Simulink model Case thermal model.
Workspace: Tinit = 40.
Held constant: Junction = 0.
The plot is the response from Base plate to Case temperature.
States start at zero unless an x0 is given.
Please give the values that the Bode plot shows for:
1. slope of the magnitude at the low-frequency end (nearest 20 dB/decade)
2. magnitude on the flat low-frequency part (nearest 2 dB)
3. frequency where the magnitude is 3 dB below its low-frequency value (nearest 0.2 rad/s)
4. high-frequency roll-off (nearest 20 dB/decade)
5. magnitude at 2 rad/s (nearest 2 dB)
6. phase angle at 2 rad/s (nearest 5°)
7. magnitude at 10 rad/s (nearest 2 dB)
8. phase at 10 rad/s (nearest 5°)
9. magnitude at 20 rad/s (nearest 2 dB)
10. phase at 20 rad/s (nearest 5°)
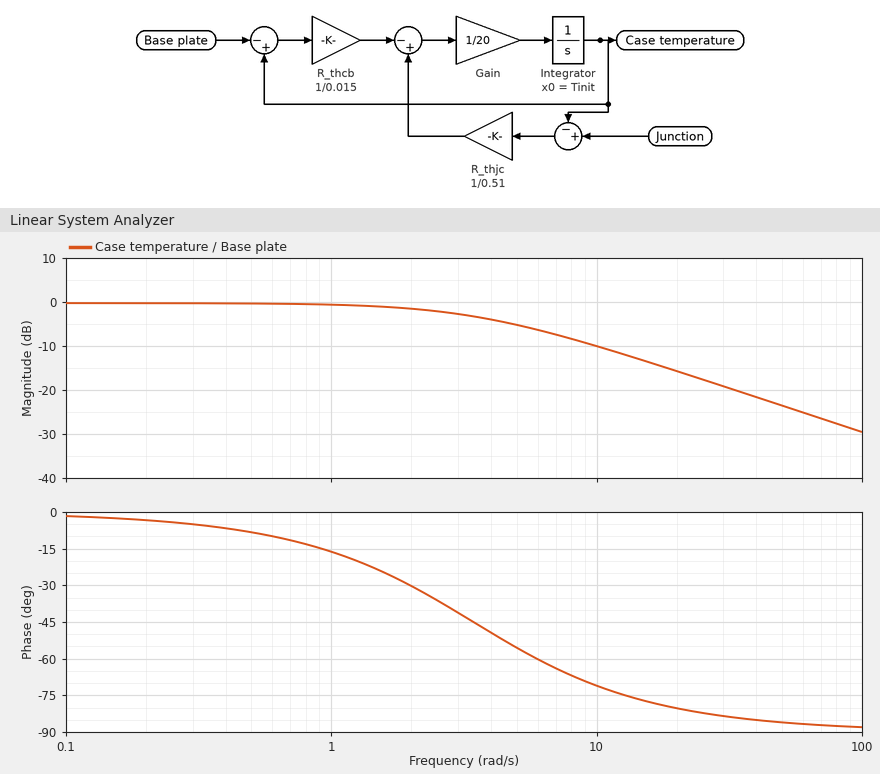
0 dB/decade
0 dB
3.4 rad/s
-20 dB/decade
-2 dB
-30°
-10 dB
-70°
-16 dB
-80°
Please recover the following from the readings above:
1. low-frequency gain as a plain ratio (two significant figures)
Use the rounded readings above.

1.0
